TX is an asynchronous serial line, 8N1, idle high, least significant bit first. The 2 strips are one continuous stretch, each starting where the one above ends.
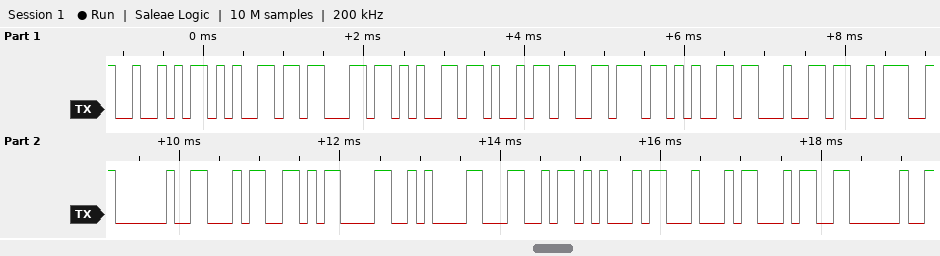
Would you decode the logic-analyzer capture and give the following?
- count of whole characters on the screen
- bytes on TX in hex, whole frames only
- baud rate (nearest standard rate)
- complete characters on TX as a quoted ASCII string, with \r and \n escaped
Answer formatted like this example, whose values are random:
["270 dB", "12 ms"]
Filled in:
["18", "52 65 63 65 69 76 65 64 3A 20 34 0D 0A 4C 45 44 34 20", "9600 baud", "\"Received: 4\\r\\nLED4 \""]
